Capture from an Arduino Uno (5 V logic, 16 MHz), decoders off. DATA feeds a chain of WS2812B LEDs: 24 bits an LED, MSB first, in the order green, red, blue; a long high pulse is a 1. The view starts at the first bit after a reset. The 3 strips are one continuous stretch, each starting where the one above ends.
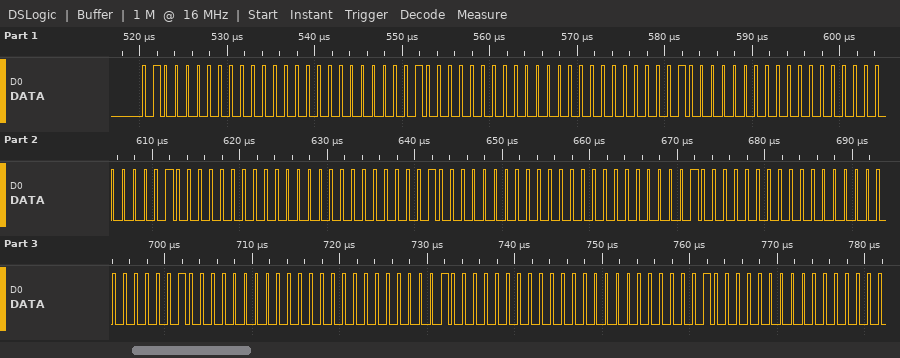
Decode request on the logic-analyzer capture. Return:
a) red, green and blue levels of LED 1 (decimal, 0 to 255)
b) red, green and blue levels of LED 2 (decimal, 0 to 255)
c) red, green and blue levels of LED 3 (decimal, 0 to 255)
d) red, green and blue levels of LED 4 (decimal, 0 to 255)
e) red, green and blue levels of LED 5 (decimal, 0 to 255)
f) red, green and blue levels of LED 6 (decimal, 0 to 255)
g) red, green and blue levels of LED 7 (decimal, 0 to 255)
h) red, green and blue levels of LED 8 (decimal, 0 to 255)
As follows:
0, 64, 0
0, 64, 0
0, 64, 0
0, 64, 0
0, 64, 0
0, 64, 0
0, 64, 0
0, 64, 0
